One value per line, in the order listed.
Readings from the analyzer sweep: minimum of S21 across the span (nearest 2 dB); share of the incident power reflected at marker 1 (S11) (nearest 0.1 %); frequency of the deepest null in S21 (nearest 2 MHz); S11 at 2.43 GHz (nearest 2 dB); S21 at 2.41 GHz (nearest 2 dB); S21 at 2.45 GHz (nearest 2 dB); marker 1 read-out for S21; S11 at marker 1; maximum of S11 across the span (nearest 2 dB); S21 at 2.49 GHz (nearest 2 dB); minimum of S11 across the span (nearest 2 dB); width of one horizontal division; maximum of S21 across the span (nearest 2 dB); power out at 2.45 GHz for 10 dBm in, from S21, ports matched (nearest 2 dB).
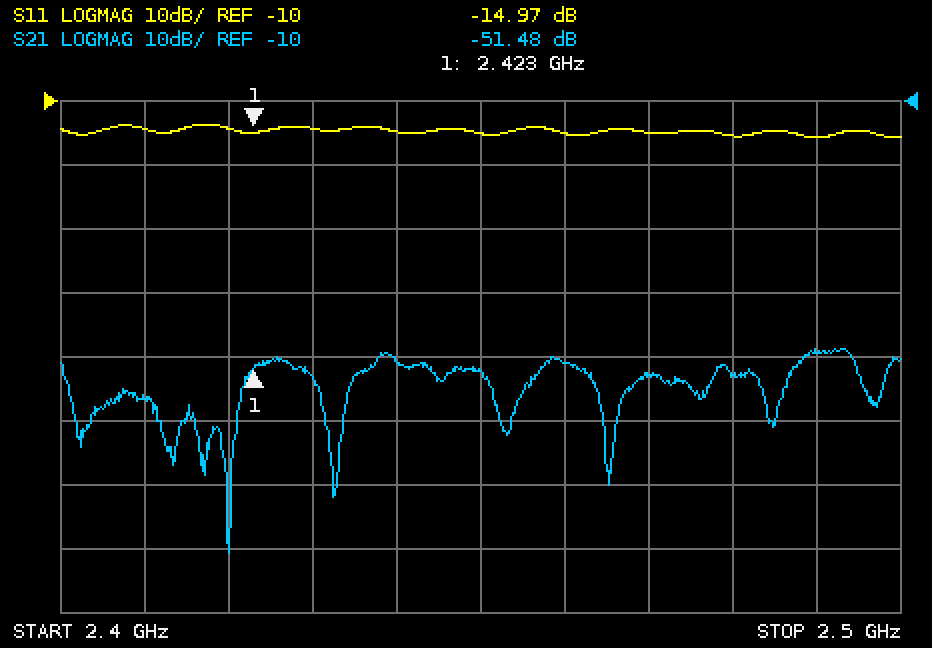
-80 dB
3.2 %
2.420 GHz
-14 dB
-56 dB
-52 dB
-51.48 dB
-14.97 dB
-14 dB
-50 dB
-16 dB
10 MHz
-48 dB
-42 dBm
